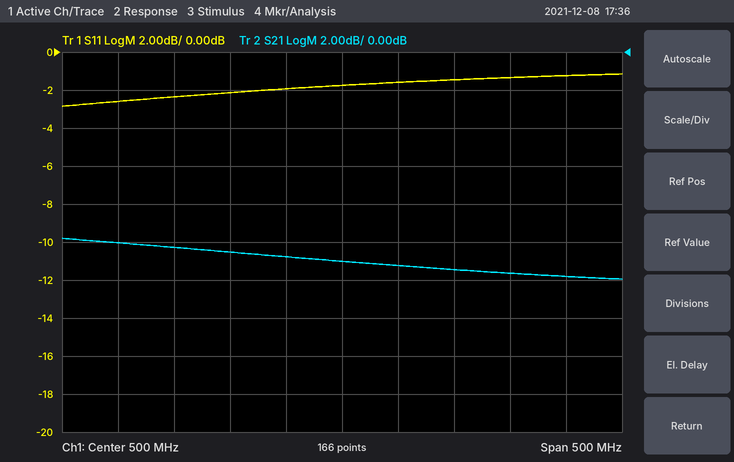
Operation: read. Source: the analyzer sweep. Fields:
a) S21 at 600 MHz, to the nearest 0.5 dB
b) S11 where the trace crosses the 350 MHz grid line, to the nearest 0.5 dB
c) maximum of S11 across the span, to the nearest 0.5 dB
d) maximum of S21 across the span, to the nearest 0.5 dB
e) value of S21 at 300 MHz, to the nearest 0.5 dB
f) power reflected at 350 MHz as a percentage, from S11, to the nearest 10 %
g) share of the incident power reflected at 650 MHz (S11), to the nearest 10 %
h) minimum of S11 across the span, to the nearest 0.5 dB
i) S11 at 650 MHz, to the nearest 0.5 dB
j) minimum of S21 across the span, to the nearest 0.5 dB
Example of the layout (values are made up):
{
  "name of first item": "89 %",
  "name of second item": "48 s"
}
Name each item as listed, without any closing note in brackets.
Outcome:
{
  "S21 at 600 MHz, to the nearest 0.5 dB": "-11.5 dB",
  "S11 where the trace crosses the 350 MHz grid line, to the nearest 0.5 dB": "-2.5 dB",
  "maximum of S11 across the span, to the nearest 0.5 dB": "-1.0 dB",
  "maximum of S21 across the span, to the nearest 0.5 dB": "-10.0 dB",
  "value of S21 at 300 MHz, to the nearest 0.5 dB": "-10.0 dB",
  "power reflected at 350 MHz as a percentage, from S11, to the nearest 10 %": "60 %",
  "share of the incident power reflected at 650 MHz (S11), to the nearest 10 %": "70 %",
  "minimum of S11 across the span, to the nearest 0.5 dB": "-3.0 dB",
  "S11 at 650 MHz, to the nearest 0.5 dB": "-1.5 dB",
  "minimum of S21 across the span, to the nearest 0.5 dB": "-12.0 dB"
}
